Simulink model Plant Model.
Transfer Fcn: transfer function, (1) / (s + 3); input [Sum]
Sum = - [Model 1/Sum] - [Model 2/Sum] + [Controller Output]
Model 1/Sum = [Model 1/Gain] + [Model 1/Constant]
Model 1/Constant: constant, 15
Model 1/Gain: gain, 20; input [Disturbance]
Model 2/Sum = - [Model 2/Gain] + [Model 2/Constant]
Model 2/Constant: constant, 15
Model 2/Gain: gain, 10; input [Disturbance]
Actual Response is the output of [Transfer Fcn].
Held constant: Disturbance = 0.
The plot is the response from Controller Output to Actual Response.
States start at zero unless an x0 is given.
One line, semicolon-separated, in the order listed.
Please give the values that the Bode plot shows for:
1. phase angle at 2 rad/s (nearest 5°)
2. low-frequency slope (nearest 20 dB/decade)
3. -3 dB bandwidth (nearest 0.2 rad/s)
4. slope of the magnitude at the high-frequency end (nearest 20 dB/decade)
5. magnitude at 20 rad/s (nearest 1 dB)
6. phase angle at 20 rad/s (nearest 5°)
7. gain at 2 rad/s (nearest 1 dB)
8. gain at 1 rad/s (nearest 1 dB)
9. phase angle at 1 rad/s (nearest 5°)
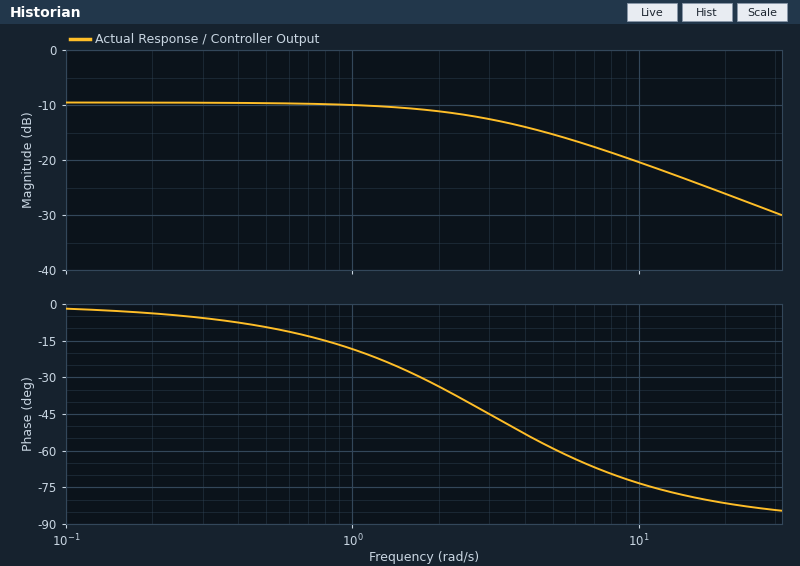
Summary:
-35°; 0 dB/decade; 3.0 rad/s; -20 dB/decade; -26 dB; -80°; -11 dB; -10 dB; -20°
